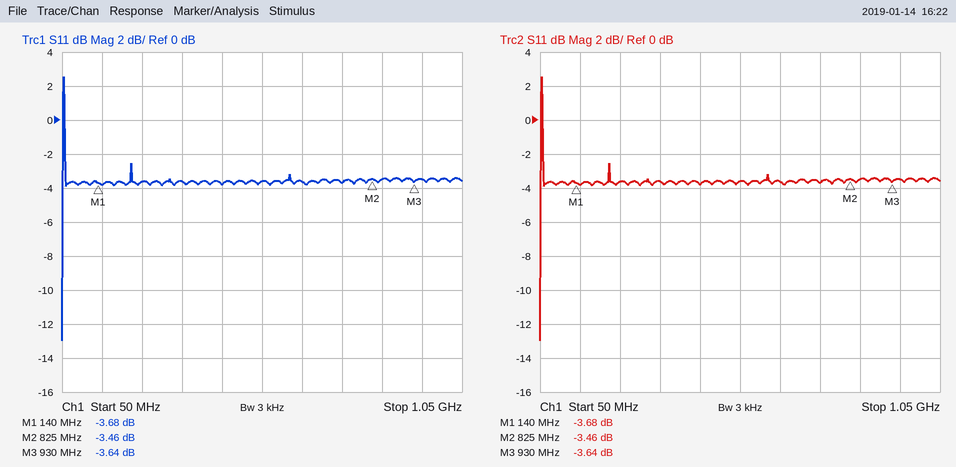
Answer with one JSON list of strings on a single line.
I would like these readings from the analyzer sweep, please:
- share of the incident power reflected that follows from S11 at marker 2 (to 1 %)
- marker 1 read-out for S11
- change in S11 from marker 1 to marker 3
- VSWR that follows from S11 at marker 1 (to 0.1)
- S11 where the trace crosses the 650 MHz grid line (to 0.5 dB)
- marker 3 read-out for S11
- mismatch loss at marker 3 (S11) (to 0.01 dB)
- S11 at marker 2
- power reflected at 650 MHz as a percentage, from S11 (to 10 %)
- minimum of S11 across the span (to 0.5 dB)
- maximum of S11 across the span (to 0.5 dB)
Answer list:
["45 %", "-3.68 dB", "0.04 dB", "4.8", "-3.5 dB", "-3.64 dB", "2.46 dB", "-3.46 dB", "40 %", "-13.0 dB", "2.5 dB"]
